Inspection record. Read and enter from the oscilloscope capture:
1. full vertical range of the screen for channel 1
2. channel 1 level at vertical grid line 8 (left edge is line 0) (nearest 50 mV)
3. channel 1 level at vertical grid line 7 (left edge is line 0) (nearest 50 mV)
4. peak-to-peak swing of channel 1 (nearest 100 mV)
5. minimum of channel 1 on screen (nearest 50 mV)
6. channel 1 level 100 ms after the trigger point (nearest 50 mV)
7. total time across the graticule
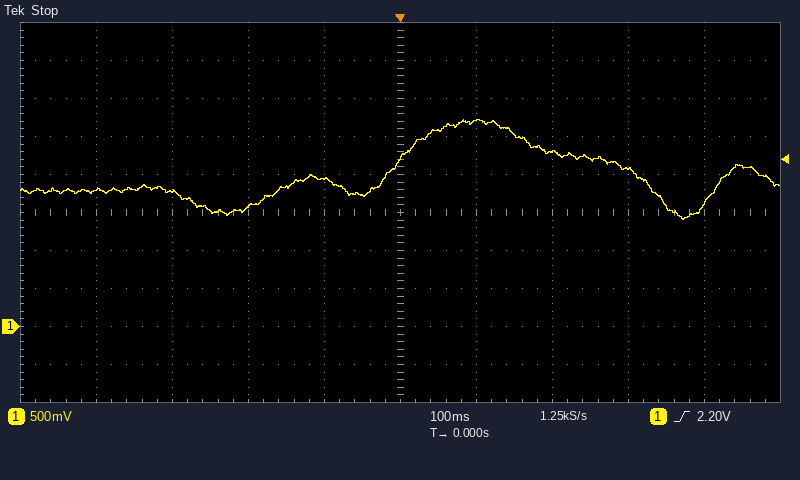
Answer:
5 V
2.05 V
2.30 V
1.30 V
1.40 V
2.70 V
1 s
